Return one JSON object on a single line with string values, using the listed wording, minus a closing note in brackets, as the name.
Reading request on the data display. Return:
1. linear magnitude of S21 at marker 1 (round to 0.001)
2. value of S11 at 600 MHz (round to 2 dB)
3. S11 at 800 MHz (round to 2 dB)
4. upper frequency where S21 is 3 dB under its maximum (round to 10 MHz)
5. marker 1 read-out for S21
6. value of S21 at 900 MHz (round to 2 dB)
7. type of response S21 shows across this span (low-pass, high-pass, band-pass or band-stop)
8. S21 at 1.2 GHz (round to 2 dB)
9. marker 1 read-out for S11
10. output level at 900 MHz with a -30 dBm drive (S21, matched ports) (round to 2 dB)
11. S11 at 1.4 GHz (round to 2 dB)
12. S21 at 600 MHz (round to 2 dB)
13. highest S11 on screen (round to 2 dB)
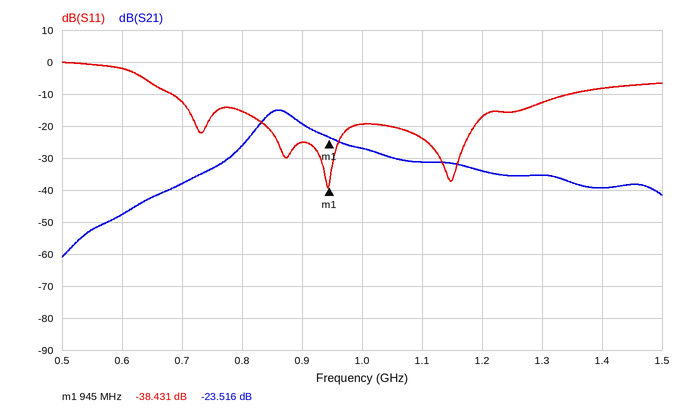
{"linear magnitude of S21 at marker 1": "0.067", "value of S11 at 600 MHz": "-2 dB", "S11 at 800 MHz": "-16 dB", "upper frequency where S21 is 3 dB under its maximum": "890 MHz", "marker 1 read-out for S21": "-23.516 dB", "value of S21 at 900 MHz": "-20 dB", "type of response S21 shows across this span": "band-pass", "S21 at 1.2 GHz": "-34 dB", "marker 1 read-out for S11": "-38.431 dB", "output level at 900 MHz with a -30 dBm drive (S21, matched ports)": "-50 dBm", "S11 at 1.4 GHz": "-8 dB", "S21 at 600 MHz": "-48 dB", "highest S11 on screen": "0 dB"}
